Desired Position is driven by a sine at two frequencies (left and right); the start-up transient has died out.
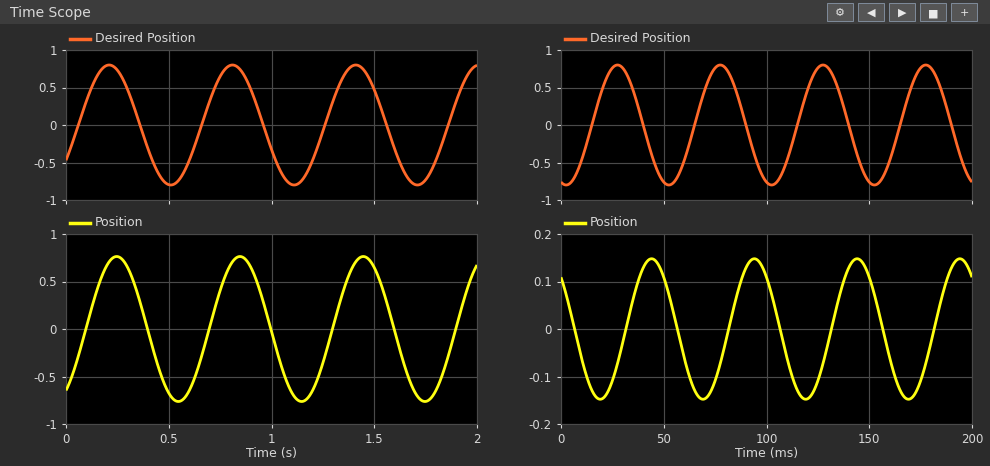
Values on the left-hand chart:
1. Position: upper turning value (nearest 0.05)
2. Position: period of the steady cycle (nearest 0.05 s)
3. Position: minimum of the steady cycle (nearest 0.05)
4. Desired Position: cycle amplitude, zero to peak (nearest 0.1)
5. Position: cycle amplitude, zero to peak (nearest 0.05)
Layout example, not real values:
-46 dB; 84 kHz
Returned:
0.75; 0.60 s; -0.75; 0.8; 0.75
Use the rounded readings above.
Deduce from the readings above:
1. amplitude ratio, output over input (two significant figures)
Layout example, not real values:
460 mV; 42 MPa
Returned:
0.94
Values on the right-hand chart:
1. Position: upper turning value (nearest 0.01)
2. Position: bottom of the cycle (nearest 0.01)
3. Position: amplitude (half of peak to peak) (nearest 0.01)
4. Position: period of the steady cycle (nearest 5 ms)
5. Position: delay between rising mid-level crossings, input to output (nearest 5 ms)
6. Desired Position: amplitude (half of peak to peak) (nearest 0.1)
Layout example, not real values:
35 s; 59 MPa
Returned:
0.15; -0.15; 0.15; 50 ms; 15 ms; 0.8
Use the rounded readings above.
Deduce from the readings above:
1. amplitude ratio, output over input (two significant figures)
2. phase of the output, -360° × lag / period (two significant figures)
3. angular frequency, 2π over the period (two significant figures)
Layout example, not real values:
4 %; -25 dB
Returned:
0.19; -110°; 0.13 rad/ms
